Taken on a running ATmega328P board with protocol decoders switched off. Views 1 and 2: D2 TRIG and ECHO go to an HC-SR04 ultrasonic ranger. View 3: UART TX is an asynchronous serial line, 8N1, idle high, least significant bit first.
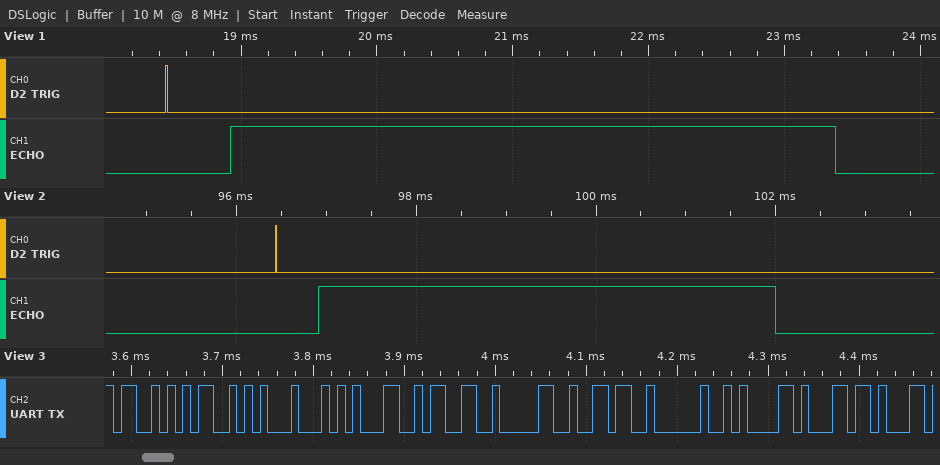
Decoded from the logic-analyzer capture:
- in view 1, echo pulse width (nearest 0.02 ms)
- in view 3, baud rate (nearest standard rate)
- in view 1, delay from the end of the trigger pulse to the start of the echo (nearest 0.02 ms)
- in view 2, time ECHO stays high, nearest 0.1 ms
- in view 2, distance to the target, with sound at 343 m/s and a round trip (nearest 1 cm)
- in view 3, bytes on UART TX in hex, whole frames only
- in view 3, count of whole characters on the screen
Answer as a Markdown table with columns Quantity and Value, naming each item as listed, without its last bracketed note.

| Quantity | Value |
|---|---|
| in view 1, echo pulse width | 4.46 ms |
| in view 3, baud rate | 115200 baud |
| in view 1, delay from the end of the trigger pulse to the start of the echo | 0.46 ms |
| in view 2, time ECHO stays high, nearest 0.1 ms | 5.1 ms |
| in view 2, distance to the target, with sound at 343 m/s and a round trip | 87 cm |
| in view 3, bytes on UART TX in hex, whole frames only | 0x53 0x53 0x44 0x31 0x33 0x30 0x36 0x20 0x61 0x6C |
| in view 3, count of whole characters on the screen | 10 |
